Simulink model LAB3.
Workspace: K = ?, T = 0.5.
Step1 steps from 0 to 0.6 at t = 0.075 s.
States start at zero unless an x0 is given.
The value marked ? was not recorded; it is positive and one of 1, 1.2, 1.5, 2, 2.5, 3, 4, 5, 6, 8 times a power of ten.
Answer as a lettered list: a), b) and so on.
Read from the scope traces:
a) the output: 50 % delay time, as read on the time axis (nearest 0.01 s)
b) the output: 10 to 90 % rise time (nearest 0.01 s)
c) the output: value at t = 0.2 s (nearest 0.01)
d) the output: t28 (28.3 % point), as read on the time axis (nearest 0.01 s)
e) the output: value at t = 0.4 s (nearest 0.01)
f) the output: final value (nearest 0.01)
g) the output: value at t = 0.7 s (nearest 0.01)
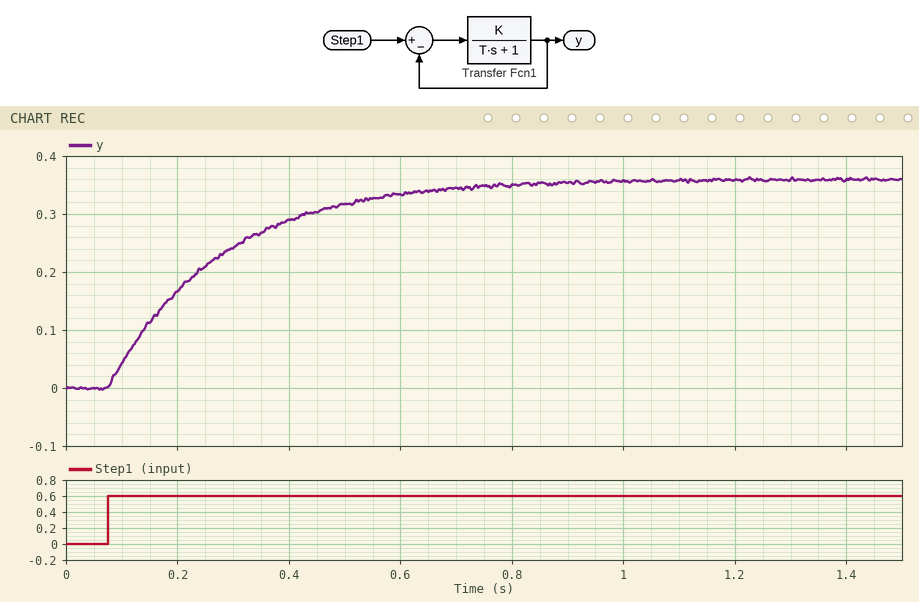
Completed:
a) 0.21 s
b) 0.44 s
c) 0.17
d) 0.14 s
e) 0.29
f) 0.36
g) 0.34
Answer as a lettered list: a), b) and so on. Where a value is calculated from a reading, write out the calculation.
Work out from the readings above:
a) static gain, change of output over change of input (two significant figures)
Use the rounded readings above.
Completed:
a) (0.36 - 0) / (0.6 - 0) = 0.60
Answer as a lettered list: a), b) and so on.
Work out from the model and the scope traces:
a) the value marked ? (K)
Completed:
a) 1.5
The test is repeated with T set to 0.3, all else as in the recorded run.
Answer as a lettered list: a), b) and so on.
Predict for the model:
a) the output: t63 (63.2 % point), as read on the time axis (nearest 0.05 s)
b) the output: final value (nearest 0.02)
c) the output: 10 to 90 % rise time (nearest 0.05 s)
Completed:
a) 0.20 s
b) 0.36
c) 0.25 s
